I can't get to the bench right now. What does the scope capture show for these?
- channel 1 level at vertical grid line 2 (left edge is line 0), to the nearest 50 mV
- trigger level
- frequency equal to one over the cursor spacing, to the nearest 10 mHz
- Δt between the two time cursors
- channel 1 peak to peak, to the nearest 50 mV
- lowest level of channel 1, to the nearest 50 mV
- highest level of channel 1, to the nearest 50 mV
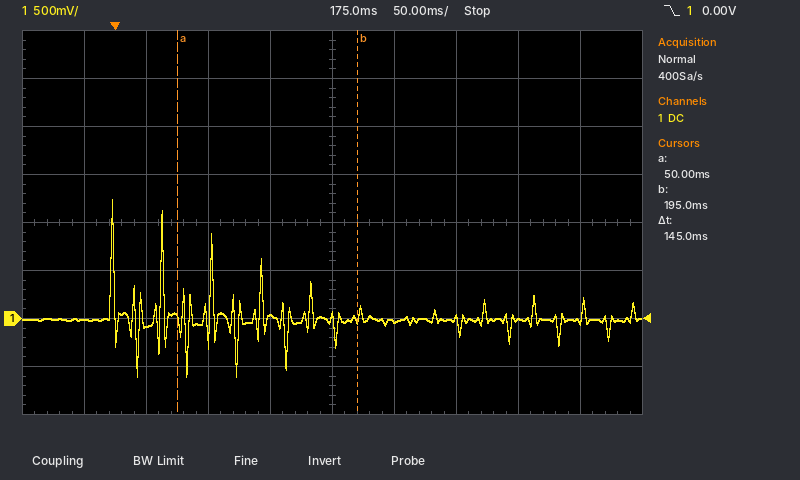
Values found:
-50 mV
0.00 V
6.90 Hz
145 ms
1.85 V
-600 mV
1.25 V
